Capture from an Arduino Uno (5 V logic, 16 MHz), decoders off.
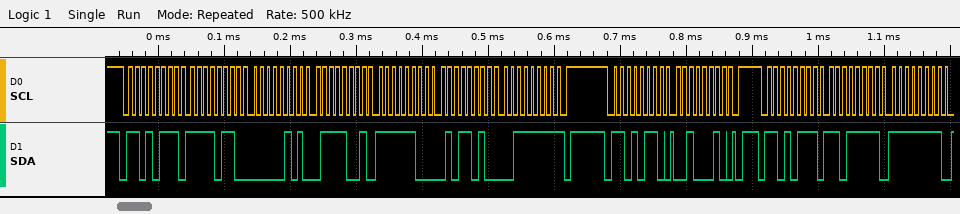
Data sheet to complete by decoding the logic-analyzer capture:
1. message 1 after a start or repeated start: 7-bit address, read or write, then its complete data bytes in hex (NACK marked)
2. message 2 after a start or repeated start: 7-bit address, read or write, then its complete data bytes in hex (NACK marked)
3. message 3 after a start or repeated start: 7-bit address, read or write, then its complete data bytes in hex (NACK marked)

0x6B read: F6 05 79 FC 5A 3F NACK
0x6B write: 22
0x6B read: DF FF
